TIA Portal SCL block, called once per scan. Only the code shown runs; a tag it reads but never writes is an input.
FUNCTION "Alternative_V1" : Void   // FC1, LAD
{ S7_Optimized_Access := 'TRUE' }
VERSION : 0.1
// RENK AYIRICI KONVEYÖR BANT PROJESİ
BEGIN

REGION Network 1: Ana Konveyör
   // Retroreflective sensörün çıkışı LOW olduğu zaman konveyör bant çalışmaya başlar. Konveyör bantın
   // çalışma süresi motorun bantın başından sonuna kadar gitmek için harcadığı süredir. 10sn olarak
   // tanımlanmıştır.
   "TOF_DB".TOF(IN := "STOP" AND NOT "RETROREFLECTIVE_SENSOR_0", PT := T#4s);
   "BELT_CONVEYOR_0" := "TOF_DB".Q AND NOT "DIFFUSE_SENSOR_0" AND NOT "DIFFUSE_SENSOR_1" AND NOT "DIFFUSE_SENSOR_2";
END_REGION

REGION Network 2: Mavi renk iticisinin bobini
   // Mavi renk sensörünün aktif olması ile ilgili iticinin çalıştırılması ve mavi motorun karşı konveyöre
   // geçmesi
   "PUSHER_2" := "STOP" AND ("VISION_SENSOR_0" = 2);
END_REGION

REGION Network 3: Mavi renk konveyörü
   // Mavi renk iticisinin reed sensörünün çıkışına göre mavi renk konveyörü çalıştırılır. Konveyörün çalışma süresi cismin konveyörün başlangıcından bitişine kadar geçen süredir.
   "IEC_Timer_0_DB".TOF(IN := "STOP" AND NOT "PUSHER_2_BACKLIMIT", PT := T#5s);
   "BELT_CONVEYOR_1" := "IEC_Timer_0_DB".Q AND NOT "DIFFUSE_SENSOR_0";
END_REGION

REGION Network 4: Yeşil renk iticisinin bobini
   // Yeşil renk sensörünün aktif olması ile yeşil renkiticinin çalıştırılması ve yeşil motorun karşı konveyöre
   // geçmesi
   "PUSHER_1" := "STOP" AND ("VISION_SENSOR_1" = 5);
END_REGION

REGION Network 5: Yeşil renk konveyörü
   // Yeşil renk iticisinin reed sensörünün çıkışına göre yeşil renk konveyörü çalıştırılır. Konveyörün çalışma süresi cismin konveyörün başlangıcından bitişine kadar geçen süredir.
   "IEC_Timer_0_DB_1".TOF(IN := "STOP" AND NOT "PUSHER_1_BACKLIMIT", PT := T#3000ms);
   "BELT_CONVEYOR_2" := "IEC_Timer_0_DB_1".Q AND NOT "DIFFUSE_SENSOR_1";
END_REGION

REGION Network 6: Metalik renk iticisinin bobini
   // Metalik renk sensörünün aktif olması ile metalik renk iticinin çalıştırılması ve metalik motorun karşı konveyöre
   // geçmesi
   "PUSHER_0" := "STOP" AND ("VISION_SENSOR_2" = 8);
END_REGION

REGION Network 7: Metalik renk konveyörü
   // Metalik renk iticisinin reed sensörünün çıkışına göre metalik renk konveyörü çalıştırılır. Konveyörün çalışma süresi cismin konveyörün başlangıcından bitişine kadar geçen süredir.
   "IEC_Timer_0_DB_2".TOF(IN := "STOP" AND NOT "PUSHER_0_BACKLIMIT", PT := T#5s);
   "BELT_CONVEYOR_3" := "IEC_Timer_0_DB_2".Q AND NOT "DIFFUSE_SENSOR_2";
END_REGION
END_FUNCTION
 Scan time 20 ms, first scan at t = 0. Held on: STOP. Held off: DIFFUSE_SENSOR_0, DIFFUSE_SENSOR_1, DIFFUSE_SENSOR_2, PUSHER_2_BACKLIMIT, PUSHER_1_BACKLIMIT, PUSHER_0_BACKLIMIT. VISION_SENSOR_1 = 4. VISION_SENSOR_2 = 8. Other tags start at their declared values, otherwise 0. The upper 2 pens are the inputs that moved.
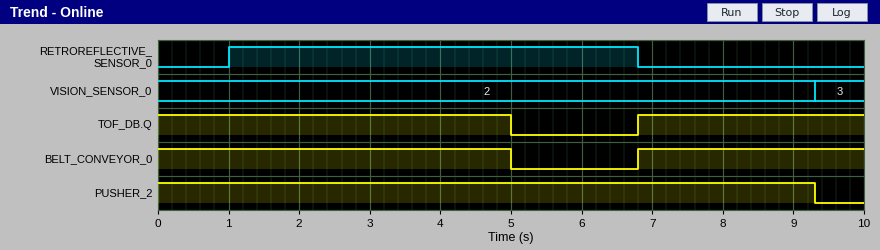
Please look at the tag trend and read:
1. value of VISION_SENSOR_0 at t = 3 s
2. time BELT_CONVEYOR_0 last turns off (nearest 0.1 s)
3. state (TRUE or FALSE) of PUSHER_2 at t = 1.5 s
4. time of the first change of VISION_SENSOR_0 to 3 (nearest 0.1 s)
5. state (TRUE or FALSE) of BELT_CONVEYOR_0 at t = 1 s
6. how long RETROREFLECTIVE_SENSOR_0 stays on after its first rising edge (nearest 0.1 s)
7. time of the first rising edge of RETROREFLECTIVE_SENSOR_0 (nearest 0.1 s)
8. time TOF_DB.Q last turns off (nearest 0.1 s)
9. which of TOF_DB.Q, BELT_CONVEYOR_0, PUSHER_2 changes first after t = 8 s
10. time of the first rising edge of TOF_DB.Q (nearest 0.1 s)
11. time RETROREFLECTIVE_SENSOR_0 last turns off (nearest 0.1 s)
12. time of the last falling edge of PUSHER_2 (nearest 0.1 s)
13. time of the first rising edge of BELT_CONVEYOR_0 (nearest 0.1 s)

2
5.0 s
TRUE
9.3 s
TRUE
5.8 s
1.0 s
5.0 s
PUSHER_2
6.8 s
6.8 s
9.3 s
6.8 s
